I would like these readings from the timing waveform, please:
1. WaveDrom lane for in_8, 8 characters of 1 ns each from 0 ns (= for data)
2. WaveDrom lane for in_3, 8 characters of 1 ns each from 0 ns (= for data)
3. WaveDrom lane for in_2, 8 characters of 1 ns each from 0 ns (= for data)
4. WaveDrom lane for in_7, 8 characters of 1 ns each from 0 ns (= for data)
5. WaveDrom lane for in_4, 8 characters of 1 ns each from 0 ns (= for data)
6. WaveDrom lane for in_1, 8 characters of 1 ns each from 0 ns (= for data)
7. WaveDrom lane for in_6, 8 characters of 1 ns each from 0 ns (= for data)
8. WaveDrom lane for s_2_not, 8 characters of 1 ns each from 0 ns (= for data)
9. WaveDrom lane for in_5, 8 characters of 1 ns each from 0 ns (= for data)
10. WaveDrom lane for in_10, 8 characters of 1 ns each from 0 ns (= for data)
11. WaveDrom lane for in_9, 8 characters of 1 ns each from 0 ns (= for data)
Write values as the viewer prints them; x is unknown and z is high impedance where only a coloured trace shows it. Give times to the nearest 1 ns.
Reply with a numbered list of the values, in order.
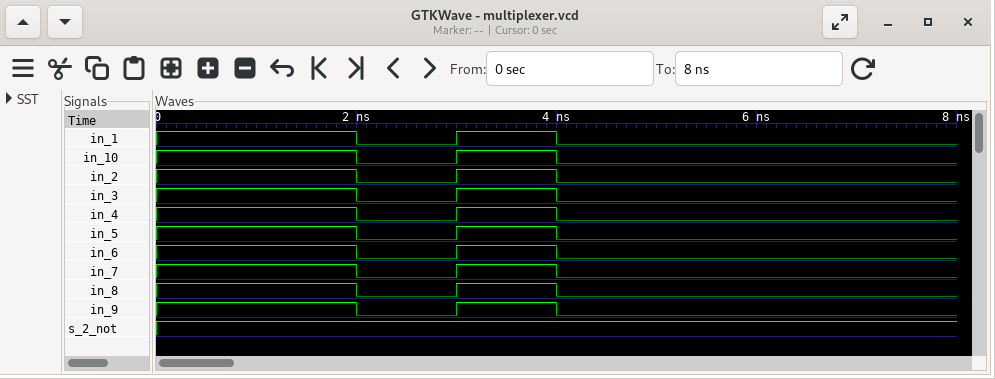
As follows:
1. {name: 'in_8', wave: '1.010...'}
2. {name: 'in_3', wave: '1.010...'}
3. {name: 'in_2', wave: '1.010...'}
4. {name: 'in_7', wave: '1.010...'}
5. {name: 'in_4', wave: '1.010...'}
6. {name: 'in_1', wave: '1.010...'}
7. {name: 'in_6', wave: '1.010...'}
8. {name: 's_2_not', wave: '1.......'}
9. {name: 'in_5', wave: '1.010...'}
10. {name: 'in_10', wave: '1.010...'}
11. {name: 'in_9', wave: '1.010...'}
